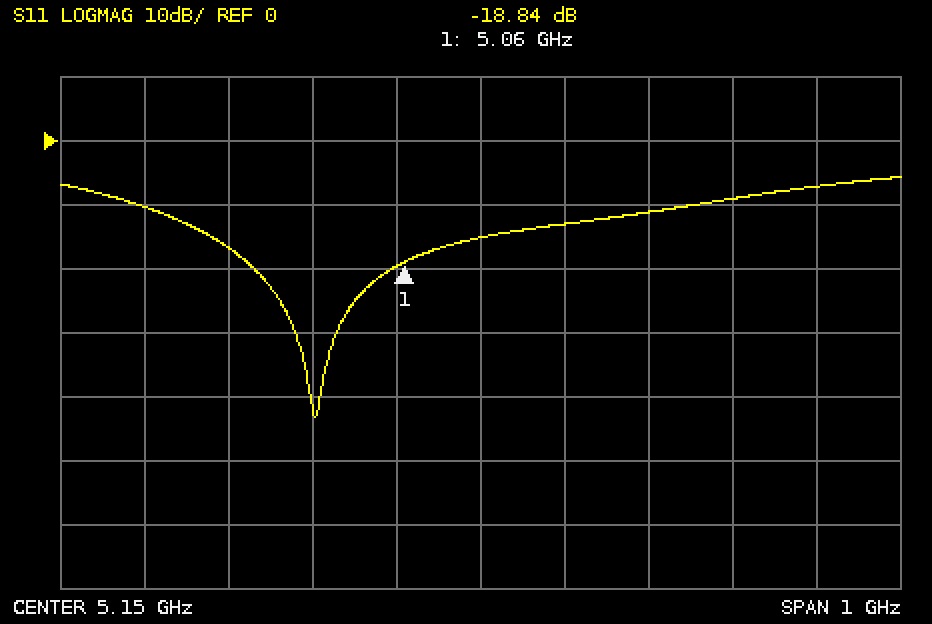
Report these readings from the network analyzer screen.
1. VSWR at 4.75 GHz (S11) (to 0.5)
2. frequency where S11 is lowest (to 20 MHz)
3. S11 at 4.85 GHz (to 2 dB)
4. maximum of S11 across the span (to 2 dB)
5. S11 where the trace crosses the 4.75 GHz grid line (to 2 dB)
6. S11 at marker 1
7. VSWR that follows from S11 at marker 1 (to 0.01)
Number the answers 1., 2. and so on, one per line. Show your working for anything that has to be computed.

1. |Γ| = 10^(-10/20) = 0.3162; VSWR = (1 + 0.3162)/(1 − 0.3162) ≈ 1.92, so 2.0 to the nearest 0.5
2. 4.96 GHz
3. -16 dB
4. -6 dB
5. -10 dB
6. -18.84 dB
7. (1 + 0.1143)/(1 − 0.1143) ≈ 1.26
